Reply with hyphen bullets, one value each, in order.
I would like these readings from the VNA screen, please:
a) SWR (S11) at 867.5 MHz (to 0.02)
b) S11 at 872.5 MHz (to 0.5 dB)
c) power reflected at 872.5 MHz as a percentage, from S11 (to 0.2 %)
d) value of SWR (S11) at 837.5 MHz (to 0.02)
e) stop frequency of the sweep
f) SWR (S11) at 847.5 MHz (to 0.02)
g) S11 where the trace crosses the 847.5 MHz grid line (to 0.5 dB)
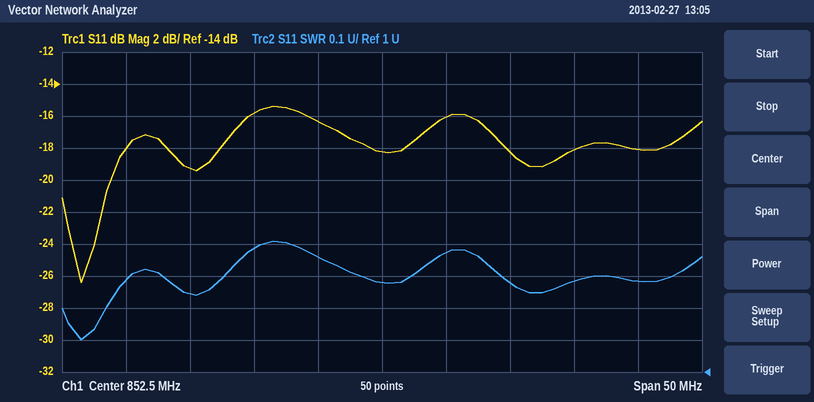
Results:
- 1.28
- -18.0 dB
- 1.6 %
- 1.24
- 877.5 MHz
- 1.36
- -16.5 dB
